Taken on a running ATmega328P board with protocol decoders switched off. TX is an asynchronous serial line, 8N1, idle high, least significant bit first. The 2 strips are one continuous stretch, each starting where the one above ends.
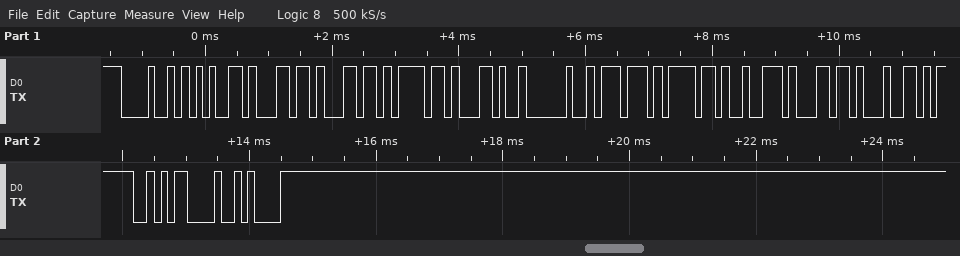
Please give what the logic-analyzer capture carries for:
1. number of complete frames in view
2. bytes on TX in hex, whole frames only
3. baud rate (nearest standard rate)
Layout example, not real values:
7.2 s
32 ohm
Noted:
15
0x48 0x65 0x6C 0x6C 0x6F 0x2C 0x20 0x77 0x6F 0x72 0x6C 0x64 0x3F 0x0D 0x0A
9600 baud
